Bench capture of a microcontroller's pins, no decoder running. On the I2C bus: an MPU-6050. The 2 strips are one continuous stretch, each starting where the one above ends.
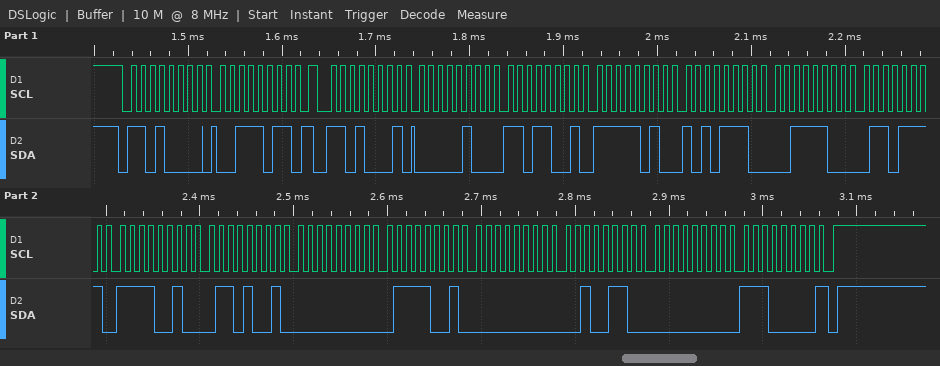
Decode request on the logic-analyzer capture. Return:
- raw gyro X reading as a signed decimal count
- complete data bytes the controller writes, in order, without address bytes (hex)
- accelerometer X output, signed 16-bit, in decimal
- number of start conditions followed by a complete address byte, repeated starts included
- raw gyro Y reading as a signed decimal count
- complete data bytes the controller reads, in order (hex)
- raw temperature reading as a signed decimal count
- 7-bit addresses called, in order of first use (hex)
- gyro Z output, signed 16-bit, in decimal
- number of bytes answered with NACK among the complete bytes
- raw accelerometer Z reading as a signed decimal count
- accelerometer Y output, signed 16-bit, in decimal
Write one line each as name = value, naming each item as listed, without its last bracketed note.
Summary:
raw gyro X reading as a signed decimal count = 121
complete data bytes the controller writes, in order, without address bytes = 3B
accelerometer X output, signed 16-bit, in decimal = 1241
number of start conditions followed by a complete address byte, repeated starts included = 2
raw gyro Y reading as a signed decimal count = 38
complete data bytes the controller reads, in order = 04 D9 FA AE 3C 6F F2 69 00 79 00 26 00 E0
raw temperature reading as a signed decimal count = -3479
7-bit addresses called, in order of first use = 0x68
gyro Z output, signed 16-bit, in decimal = 224
number of bytes answered with NACK among the complete bytes = 1
raw accelerometer Z reading as a signed decimal count = 15471
accelerometer Y output, signed 16-bit, in decimal = -1362
